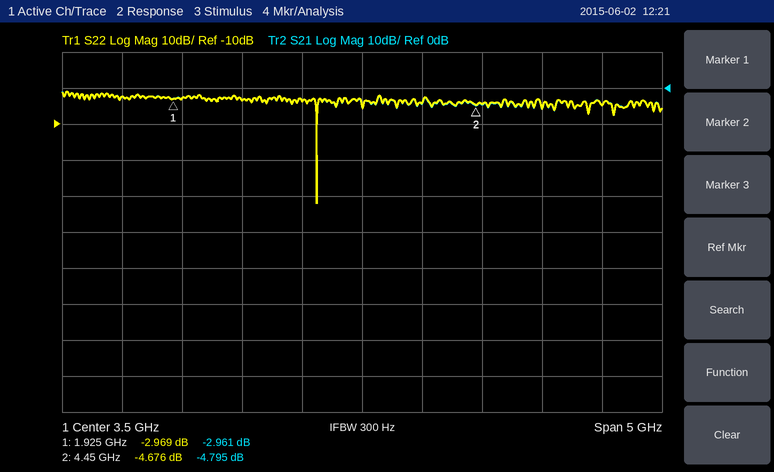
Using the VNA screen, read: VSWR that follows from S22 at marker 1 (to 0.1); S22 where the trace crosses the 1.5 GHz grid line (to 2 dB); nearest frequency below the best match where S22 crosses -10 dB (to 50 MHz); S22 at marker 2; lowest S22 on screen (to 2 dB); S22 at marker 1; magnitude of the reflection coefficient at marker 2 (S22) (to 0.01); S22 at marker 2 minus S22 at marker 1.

5.9
-2 dB
3.10 GHz
-4.676 dB
-32 dB
-2.969 dB
0.58
-1.707 dB
